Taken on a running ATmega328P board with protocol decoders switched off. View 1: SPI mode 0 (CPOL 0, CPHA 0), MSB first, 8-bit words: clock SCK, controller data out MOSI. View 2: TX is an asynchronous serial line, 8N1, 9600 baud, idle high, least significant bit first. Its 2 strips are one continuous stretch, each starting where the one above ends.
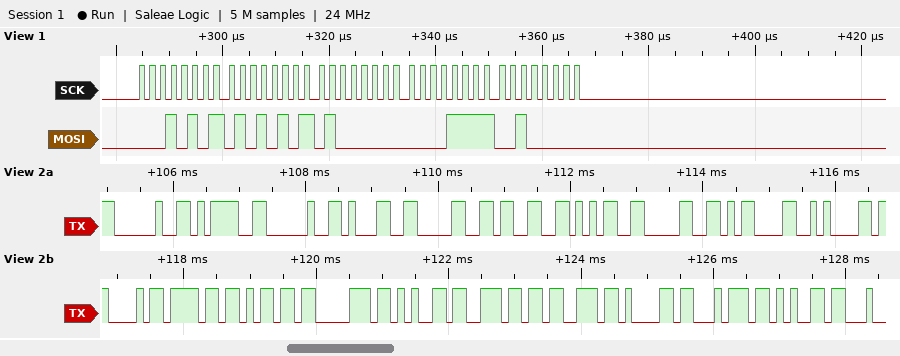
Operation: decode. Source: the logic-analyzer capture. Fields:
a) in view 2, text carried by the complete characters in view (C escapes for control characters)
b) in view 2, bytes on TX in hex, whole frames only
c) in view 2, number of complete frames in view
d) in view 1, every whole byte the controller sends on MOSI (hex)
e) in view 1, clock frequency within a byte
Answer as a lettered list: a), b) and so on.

a) " = 10350\r\nCompensate"
b) 20 3D 20 31 30 33 35 30 0D 0A 43 6F 6D 70 65 6E 73 61 74 65
c) 20
d) 15 55 40 0F 20
e) 500 kHz
